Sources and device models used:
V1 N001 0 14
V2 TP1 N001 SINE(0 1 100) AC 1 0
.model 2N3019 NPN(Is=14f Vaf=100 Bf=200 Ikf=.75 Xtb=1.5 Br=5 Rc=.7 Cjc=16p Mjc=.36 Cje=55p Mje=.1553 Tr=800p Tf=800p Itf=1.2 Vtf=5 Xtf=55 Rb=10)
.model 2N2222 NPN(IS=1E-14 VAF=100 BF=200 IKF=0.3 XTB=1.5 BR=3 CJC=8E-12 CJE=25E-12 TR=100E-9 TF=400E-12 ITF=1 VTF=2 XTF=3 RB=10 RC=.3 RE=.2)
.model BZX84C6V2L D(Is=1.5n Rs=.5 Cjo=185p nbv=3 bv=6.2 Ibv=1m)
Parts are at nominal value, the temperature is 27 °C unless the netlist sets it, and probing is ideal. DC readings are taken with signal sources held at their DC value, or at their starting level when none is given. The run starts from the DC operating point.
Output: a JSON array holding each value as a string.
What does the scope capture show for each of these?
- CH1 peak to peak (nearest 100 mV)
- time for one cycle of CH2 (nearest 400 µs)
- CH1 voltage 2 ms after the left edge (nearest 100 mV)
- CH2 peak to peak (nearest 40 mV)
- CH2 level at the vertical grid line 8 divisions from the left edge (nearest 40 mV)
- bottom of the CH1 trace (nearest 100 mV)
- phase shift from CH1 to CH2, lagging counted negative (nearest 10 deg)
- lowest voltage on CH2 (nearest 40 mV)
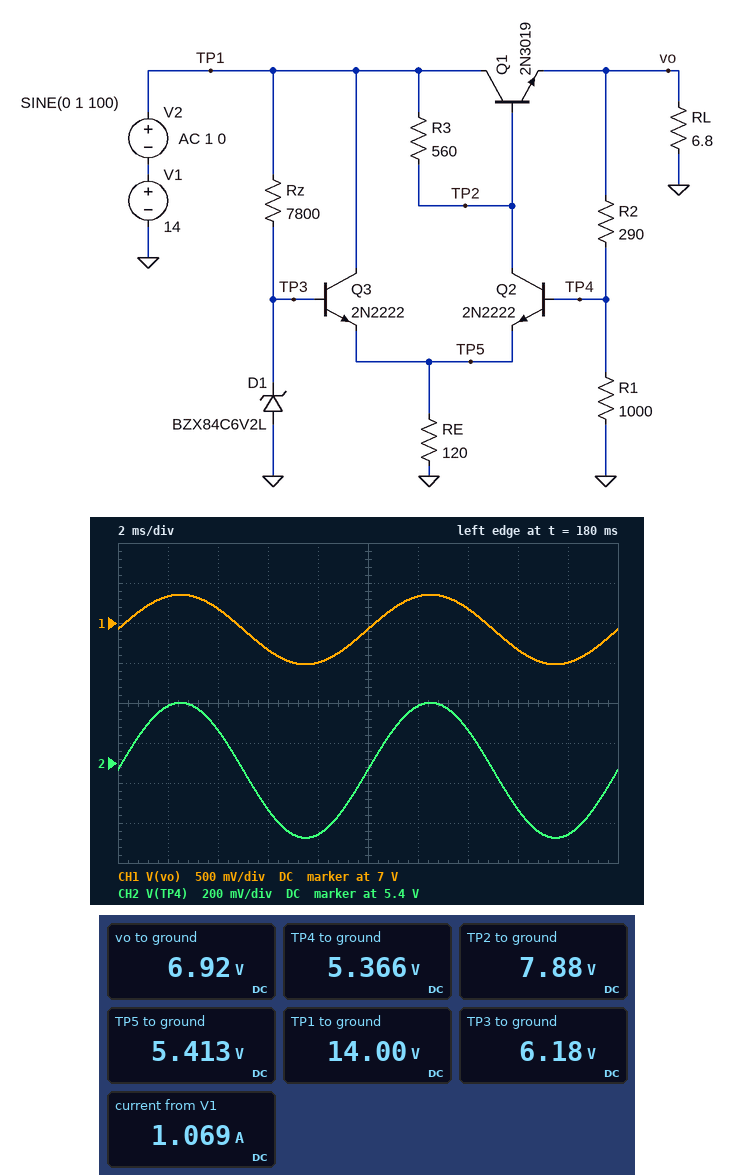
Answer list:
["900 mV", "10.0 ms", "7.3 V", "680 mV", "5.16 V", "6.5 V", "0 deg", "5.04 V"]
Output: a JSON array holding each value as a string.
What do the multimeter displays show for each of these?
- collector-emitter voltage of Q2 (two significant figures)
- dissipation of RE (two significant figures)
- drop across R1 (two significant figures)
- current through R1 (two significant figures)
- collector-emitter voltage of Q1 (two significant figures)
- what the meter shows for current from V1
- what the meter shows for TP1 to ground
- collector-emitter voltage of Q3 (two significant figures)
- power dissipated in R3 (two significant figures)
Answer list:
["2.5 V", "240 mW", "5.4 V", "5.4 mA", "7.1 V", "1.069 A", "14.00 V", "8.6 V", "67 mW"]
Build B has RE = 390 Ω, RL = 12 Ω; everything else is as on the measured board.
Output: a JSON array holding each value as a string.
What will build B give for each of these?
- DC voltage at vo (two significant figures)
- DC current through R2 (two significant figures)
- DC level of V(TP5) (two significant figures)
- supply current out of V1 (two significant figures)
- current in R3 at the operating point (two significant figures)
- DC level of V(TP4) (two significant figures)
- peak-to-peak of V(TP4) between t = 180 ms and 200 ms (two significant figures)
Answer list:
["8.0 V", "6.2 mA", "5.5 V", "680 mA", "9.2 mA", "6.2 V", "63 mV"]
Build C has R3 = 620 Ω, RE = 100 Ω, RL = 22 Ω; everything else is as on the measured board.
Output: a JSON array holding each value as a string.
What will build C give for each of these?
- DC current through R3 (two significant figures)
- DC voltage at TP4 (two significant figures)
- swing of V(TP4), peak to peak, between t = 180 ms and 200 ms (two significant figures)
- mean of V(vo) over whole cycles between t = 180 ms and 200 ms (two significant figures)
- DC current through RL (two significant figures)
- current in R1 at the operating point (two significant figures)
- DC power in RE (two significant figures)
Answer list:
["8.5 mA", "6.1 V", "47 mV", "7.9 V", "360 mA", "6.1 mA", "290 mW"]
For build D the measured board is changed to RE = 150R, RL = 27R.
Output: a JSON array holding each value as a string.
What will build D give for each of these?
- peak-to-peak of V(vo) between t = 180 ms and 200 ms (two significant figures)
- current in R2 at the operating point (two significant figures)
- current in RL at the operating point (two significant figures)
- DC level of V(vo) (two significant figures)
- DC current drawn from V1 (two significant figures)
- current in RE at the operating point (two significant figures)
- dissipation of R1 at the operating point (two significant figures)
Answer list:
["61 mV", "6.2 mA", "290 mA", "7.9 V", "340 mA", "36 mA", "38 mW"]
